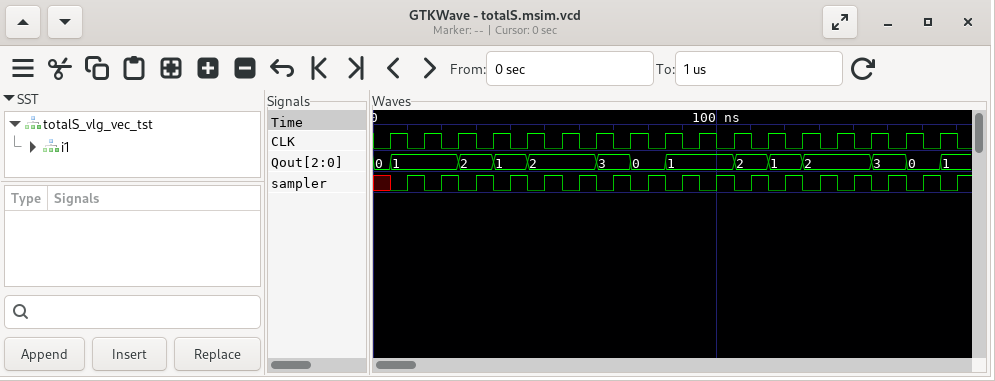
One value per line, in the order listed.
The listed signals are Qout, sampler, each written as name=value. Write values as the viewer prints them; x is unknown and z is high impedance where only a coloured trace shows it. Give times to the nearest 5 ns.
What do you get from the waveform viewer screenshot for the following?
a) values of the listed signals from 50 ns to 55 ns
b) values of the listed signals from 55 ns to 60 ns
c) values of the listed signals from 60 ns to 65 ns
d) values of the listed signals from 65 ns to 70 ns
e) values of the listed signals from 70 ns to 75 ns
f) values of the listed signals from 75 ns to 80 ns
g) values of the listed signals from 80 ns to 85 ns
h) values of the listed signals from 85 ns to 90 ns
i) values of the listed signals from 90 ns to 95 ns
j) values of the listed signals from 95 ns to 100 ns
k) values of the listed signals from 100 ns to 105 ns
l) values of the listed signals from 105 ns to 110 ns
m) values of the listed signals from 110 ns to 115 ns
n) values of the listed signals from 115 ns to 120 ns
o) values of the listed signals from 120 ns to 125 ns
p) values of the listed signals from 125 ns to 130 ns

Qout=2, sampler=1
Qout=2, sampler=0
Qout=2, sampler=1
Qout=3, sampler=0
Qout=3, sampler=1
Qout=0, sampler=0
Qout=0, sampler=1
Qout=1, sampler=0
Qout=1, sampler=1
Qout=1, sampler=0
Qout=1, sampler=1
Qout=2, sampler=0
Qout=2, sampler=1
Qout=1, sampler=0
Qout=1, sampler=1
Qout=2, sampler=0
